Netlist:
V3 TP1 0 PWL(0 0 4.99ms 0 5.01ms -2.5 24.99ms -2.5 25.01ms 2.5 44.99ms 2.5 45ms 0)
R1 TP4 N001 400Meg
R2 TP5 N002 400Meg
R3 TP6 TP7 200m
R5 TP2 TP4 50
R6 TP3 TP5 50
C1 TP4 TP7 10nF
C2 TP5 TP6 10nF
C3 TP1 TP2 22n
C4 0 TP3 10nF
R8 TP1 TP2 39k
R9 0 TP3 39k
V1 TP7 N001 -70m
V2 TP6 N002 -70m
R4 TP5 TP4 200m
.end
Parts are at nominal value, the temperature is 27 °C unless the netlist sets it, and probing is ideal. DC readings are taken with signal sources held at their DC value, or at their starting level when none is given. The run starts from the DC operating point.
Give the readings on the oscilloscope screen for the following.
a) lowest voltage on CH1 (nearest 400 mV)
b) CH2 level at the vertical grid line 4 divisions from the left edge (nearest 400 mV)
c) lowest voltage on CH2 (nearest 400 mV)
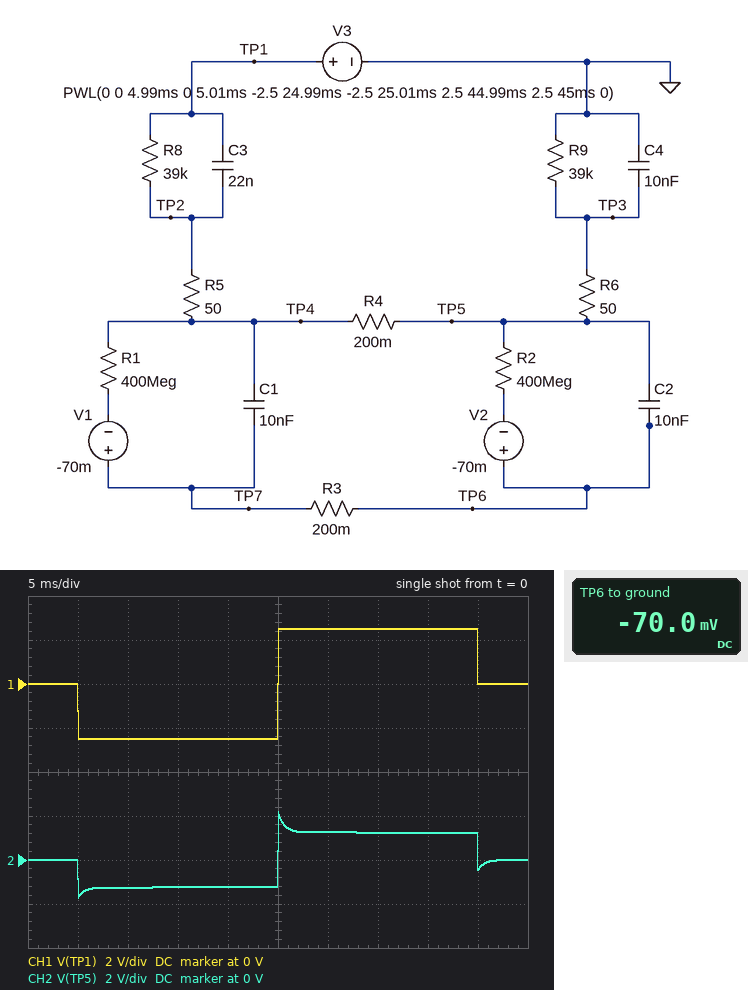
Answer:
-2.4 V
-1.2 V
-1.6 V
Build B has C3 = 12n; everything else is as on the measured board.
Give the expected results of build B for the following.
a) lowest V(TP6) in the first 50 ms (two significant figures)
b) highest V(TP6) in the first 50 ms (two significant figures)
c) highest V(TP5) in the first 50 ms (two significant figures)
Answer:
-1.4 V
1.4 V
1.5 V
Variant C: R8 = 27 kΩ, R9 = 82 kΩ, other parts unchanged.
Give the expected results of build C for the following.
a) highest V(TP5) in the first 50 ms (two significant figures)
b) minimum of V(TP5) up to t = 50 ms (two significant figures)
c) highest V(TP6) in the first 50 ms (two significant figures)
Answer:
1.9 V
-1.9 V
1.8 V
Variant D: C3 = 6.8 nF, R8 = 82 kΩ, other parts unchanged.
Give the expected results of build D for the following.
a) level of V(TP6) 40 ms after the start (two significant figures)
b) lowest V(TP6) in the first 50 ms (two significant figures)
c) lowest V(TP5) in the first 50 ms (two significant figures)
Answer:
740 mV
-1.1 V
-1.0 V
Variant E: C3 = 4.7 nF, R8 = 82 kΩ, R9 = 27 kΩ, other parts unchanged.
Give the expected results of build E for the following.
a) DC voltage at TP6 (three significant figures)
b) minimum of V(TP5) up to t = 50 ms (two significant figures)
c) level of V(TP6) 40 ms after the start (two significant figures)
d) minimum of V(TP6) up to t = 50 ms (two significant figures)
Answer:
-70.0 mV
-800 mV
550 mV
-870 mV
